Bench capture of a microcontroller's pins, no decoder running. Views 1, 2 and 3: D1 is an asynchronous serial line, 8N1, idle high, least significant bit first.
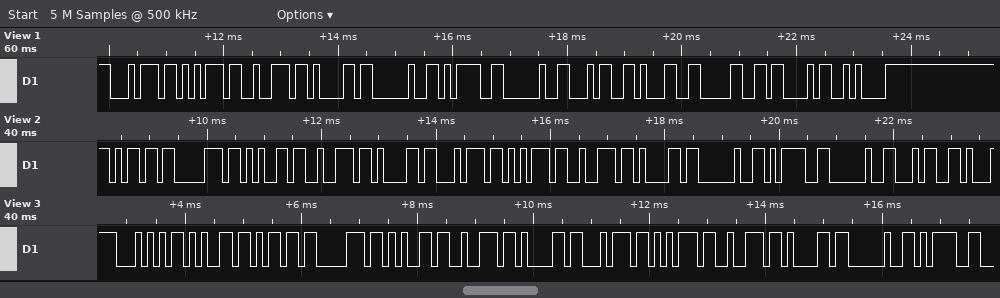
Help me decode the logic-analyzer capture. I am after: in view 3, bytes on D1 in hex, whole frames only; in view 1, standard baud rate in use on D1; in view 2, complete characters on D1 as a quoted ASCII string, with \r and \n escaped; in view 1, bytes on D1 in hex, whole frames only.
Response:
54 65 6D 70 65 72 61 74 75 72 61 20 3D
9600 baud
"mperatura = 4"
74 75 72 61 20 3D 20 34 31 30 43 0A
